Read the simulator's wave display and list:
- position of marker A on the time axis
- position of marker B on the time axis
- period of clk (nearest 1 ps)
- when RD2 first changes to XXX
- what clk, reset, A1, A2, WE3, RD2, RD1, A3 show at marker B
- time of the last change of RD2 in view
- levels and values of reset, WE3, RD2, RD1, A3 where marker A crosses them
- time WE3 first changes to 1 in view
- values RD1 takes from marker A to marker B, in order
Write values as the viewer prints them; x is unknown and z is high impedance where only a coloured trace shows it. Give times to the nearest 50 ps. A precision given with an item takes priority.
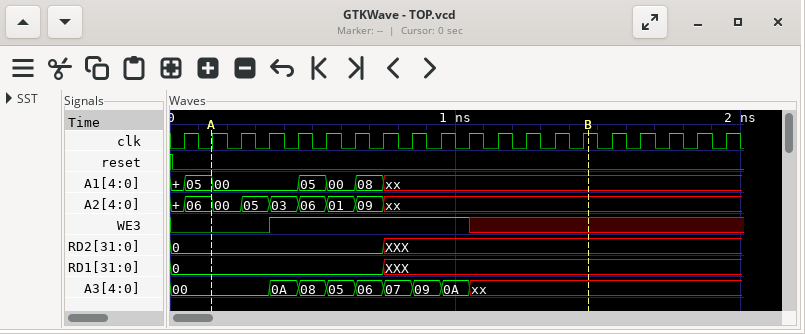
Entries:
150 ps
1450 ps
100 ps
750 ps
clk=1, reset=0, A1=xx, A2=xx, WE3=x, RD2=XXX, RD1=XXX, A3=xx
750 ps
reset=0, WE3=0, RD2=0, RD1=0, A3=00
350 ps
0, XXX
